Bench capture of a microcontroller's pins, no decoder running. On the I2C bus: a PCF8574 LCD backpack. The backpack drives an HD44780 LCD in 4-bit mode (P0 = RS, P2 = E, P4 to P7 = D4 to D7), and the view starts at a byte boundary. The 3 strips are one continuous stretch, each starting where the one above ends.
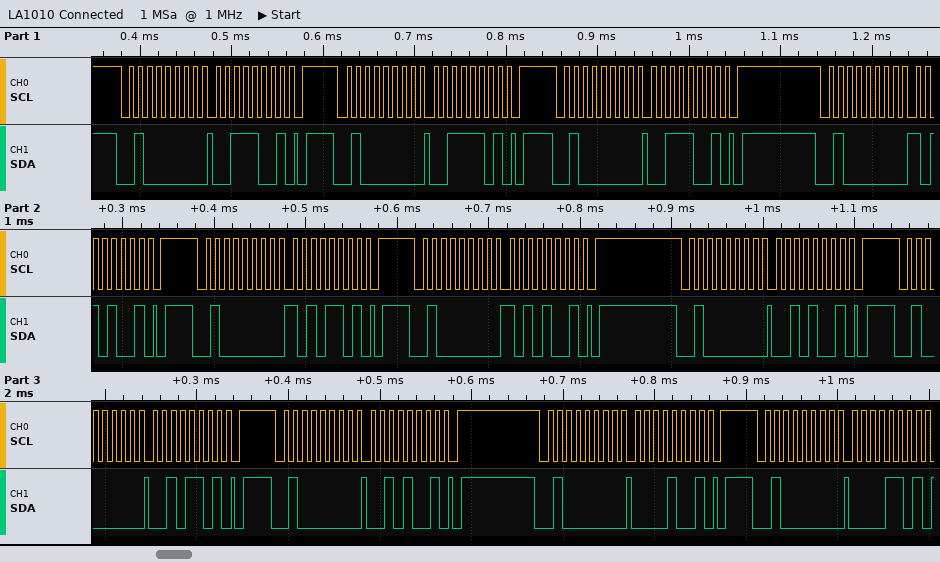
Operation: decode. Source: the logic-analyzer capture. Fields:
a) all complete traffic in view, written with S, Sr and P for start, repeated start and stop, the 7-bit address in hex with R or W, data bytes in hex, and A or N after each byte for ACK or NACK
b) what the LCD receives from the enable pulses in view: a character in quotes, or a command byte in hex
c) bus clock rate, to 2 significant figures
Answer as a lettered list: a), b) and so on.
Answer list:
a) S 20W A 39 A P S 20W A 3D A P S 20W A 39 A P S 20W A A9 A P S 20W A AD A P S 20W A A9 A P S 20W A 29 A P S 20W A 2D A P S 20W A 29 A P S 20W A 09 A P S 20W A 0D A
b) ':'
c) 100 kHz
